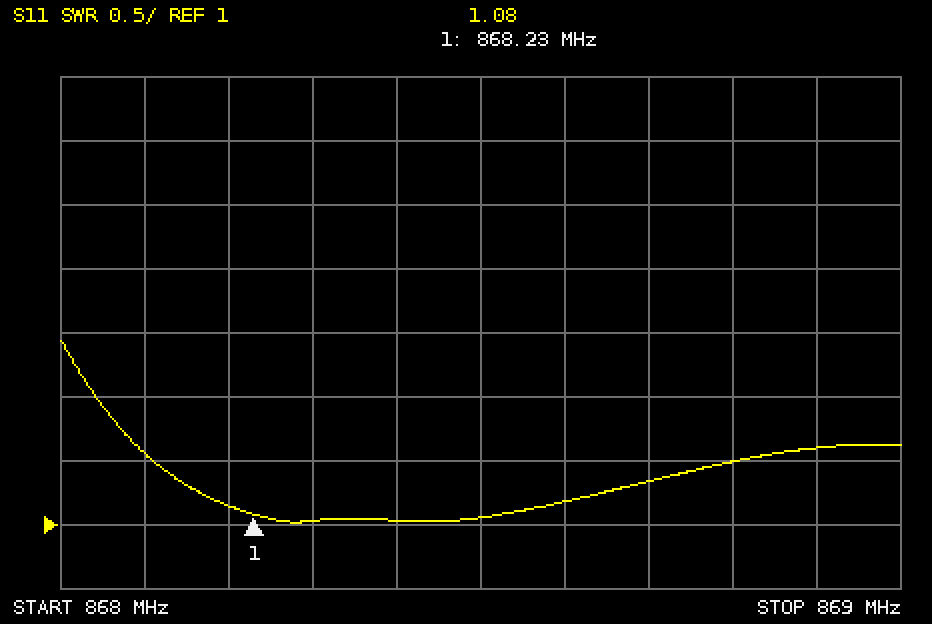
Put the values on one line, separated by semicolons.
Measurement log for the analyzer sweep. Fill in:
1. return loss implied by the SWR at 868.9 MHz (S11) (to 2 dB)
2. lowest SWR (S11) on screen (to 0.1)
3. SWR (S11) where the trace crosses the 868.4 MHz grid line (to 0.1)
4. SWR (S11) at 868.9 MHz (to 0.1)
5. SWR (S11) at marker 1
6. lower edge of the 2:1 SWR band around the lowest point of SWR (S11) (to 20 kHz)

12 dB; 1.0; 1.0; 1.6; 1.08; 868.04 MHz
